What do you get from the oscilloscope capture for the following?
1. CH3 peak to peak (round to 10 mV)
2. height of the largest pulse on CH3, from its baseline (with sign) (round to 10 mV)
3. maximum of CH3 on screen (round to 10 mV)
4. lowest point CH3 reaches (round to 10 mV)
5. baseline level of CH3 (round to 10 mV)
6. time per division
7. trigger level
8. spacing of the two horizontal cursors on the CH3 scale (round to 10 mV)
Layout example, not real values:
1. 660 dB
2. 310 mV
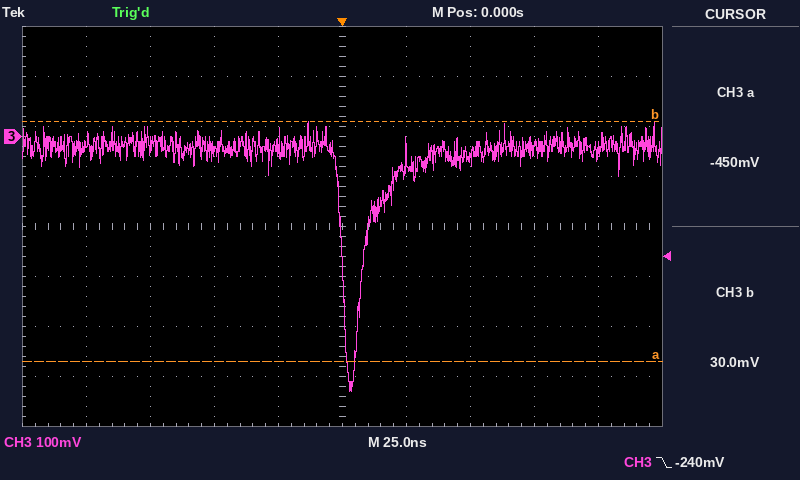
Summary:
1. 540 mV
2. -490 mV
3. 30 mV
4. -510 mV
5. -20 mV
6. 25 ns
7. -240 mV
8. 480 mV
